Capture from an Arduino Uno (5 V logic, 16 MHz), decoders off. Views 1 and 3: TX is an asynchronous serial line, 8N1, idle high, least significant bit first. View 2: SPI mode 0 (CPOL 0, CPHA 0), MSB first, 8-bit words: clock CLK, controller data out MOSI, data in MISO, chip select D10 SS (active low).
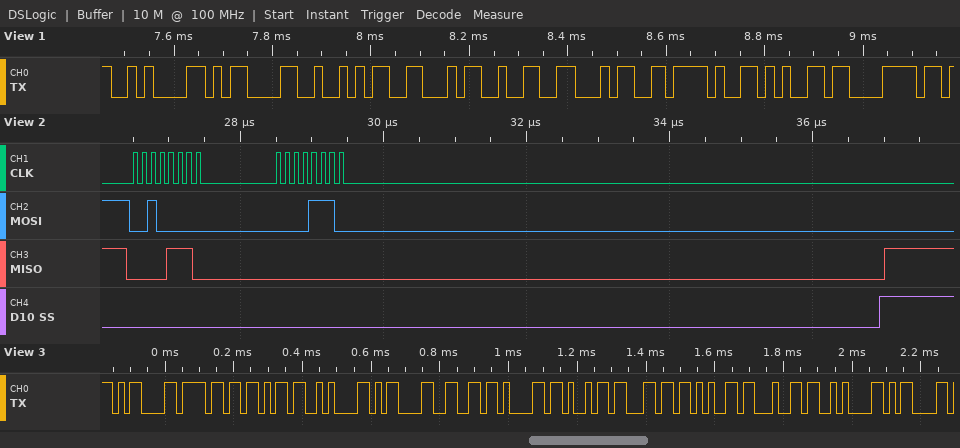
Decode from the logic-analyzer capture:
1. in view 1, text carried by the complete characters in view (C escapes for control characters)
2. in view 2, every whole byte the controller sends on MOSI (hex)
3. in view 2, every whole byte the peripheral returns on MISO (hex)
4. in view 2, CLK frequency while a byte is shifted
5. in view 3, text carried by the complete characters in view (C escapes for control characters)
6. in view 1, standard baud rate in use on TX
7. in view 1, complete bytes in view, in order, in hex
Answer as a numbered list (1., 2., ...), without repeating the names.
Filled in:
1. "\n\rRF24/ex"
2. 20 0E
3. 0E 00
4. 8 MHz
5. "\rok\n\rfailed\n\r"
6. 57600 baud
7. 0A 0D 52 46 32 34 2F 65 78
